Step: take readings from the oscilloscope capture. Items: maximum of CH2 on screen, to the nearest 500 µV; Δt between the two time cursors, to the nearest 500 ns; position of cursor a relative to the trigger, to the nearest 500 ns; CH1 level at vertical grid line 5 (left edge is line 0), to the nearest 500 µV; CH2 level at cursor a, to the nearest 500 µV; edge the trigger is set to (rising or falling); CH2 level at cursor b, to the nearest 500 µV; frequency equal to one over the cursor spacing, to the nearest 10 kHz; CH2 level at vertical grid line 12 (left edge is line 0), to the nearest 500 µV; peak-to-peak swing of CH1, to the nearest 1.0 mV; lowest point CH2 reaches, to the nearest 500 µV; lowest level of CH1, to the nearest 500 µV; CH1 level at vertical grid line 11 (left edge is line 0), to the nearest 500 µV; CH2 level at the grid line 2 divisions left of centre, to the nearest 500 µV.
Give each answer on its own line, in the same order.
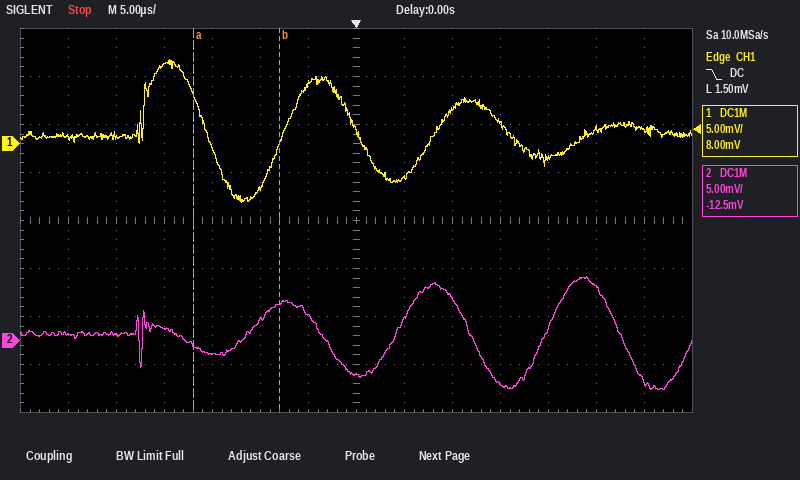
6.5 mV
9.0 µs
-17.0 µs
-4.5 mV
-500 µV
falling
4.0 mV
110 kHz
5.5 mV
15.0 mV
-5.0 mV
-6.0 mV
-1.5 mV
2.0 mV
